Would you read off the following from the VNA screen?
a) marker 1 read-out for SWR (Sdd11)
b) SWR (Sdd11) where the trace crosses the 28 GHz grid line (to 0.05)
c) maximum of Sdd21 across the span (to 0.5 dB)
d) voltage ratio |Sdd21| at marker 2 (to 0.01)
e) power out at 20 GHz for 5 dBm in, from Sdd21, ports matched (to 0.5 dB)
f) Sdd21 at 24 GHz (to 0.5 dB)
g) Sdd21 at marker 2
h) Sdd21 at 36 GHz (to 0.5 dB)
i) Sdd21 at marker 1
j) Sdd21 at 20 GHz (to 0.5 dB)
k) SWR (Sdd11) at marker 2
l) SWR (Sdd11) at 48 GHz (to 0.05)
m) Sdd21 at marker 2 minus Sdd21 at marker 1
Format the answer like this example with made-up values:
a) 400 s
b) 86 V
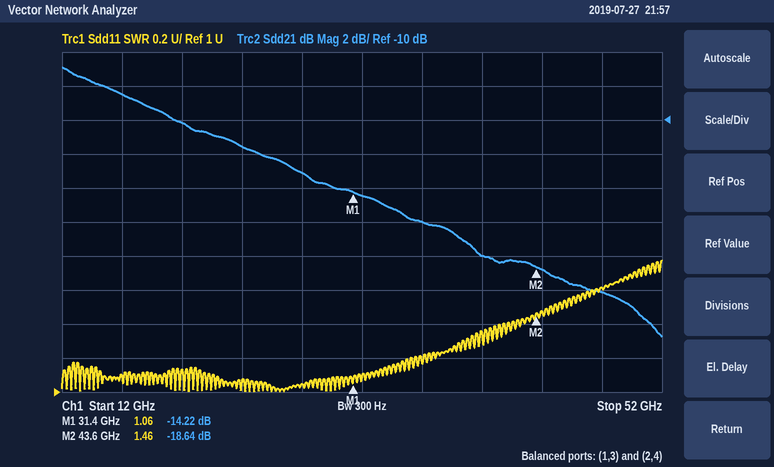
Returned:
a) 1.06
b) 1.05
c) -7.0 dB
d) 0.12
e) -5.0 dBm
f) -11.5 dB
g) -18.64 dB
h) -16.0 dB
i) -14.22 dB
j) -10.0 dB
k) 1.46
l) 1.60
m) -4.42 dB
